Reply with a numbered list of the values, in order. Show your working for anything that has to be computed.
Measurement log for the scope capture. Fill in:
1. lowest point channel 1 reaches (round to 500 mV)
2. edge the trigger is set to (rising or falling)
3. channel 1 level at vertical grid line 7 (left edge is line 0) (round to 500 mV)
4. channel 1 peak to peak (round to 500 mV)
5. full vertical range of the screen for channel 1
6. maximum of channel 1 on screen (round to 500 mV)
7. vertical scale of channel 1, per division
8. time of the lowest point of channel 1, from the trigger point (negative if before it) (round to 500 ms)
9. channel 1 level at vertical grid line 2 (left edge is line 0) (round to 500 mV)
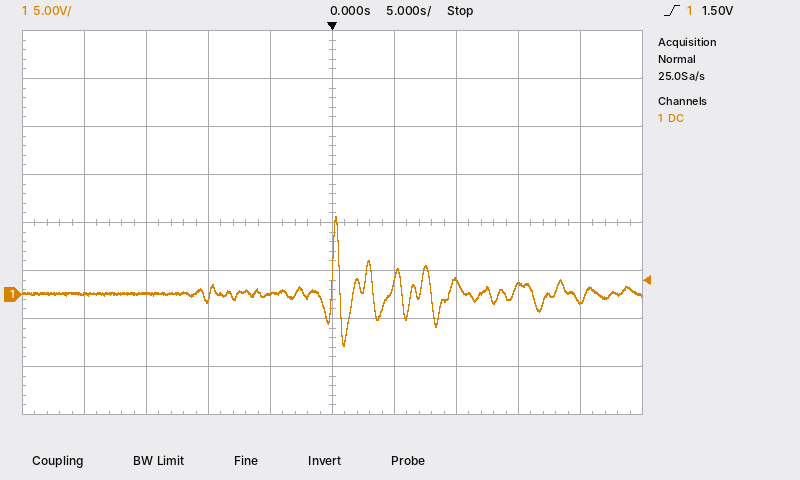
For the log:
1. -5.5 V
2. rising
3. 1.5 V
4. 8.0 V − (-5.5 V) = 13.5 V
5. 40 V
6. 8.0 V
7. 5 V
8. +1.0 s
9. 0.0 V
